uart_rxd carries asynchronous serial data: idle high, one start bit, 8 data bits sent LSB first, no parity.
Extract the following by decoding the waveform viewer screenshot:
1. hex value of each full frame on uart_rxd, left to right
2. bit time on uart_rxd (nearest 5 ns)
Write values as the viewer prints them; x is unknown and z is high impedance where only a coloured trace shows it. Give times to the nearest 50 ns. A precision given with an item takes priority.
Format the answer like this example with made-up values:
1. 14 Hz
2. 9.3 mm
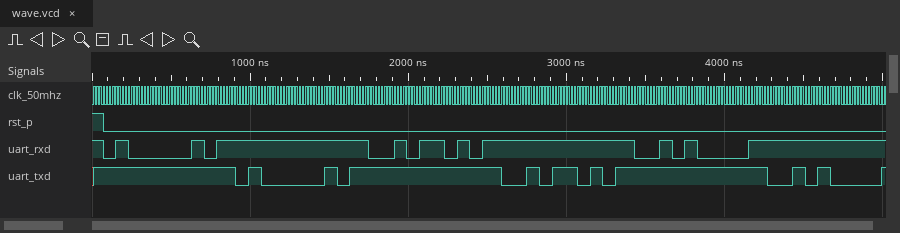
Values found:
1. 41, 5A, 0A
2. 80 ns
